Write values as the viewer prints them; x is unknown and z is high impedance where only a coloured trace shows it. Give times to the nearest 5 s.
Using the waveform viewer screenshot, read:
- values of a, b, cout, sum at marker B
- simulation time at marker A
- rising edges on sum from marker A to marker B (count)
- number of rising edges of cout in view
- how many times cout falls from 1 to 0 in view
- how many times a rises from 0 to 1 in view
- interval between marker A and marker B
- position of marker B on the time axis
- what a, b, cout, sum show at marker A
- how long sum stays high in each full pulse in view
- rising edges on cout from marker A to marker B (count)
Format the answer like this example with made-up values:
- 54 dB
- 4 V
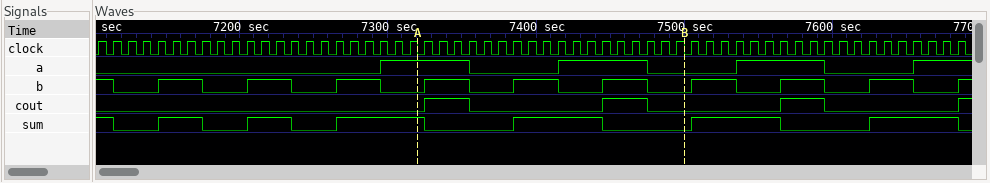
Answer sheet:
- a=0, b=0, cout=0, sum=0
- 7320 s
- 1
- 4
- 3
- 4
- 180 s
- 7500 s
- a=1, b=0, cout=0, sum=1
- 30 s, 30 s, 60 s, 60 s, 60 s, 60 s
- 2
